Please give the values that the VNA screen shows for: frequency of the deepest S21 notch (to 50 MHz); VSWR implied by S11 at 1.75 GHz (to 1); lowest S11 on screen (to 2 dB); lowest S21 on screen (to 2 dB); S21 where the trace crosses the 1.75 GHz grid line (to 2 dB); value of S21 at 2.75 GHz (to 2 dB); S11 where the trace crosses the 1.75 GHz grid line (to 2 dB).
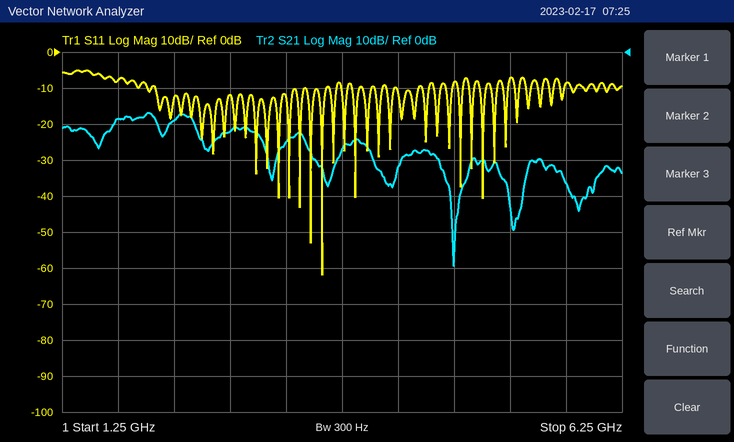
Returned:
4.75 GHz
2
-62 dB
-60 dB
-18 dB
-22 dB
-8 dB
